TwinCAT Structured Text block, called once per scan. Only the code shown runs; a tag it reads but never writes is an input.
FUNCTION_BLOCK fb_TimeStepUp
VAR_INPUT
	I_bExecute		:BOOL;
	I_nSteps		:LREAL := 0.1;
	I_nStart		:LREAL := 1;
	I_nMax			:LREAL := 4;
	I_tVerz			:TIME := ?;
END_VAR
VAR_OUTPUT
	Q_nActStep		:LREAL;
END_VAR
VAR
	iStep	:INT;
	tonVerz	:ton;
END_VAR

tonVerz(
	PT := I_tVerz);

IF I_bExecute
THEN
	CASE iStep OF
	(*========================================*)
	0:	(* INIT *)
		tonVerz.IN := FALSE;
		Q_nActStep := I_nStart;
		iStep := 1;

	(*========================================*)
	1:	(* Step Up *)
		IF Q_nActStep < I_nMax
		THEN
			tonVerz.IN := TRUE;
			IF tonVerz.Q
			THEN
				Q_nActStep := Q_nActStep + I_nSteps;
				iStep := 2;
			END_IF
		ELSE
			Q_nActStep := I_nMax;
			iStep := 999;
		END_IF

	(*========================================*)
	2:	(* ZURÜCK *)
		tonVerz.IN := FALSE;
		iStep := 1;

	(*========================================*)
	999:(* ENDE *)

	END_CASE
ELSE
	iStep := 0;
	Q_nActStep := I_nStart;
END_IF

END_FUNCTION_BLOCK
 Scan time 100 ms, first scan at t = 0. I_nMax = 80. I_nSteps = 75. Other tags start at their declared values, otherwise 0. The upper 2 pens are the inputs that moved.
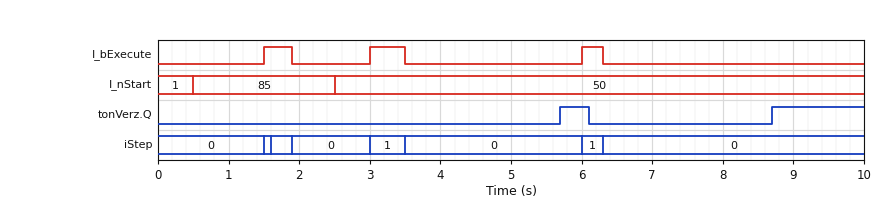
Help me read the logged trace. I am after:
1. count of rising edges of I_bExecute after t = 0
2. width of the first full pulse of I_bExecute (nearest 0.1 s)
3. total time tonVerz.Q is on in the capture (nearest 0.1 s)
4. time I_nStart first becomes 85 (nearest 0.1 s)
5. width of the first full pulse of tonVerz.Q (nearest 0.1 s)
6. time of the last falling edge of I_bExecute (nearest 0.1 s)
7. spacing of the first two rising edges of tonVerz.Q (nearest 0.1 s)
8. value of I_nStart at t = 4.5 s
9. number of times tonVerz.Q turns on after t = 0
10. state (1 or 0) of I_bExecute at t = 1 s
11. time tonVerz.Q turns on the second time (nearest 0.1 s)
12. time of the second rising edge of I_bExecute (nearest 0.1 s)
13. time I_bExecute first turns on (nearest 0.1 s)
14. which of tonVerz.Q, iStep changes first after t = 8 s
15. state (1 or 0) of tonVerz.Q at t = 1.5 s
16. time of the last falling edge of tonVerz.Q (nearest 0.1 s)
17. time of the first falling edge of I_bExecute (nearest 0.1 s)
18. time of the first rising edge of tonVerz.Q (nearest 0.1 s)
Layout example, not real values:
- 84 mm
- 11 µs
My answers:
- 3
- 0.4 s
- 1.7 s
- 0.5 s
- 0.4 s
- 6.3 s
- 3.0 s
- 50
- 2
- 0
- 8.7 s
- 3.0 s
- 1.5 s
- tonVerz.Q
- 0
- 6.1 s
- 1.9 s
- 5.7 s
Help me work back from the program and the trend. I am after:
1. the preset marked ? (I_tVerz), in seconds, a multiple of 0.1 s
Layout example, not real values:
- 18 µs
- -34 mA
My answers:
- 2.5 s
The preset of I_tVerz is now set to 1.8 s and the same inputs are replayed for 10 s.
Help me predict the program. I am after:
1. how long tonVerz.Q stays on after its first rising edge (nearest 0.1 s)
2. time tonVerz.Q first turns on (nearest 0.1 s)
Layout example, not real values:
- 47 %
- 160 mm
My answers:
- 1.1 s
- 5.0 s
